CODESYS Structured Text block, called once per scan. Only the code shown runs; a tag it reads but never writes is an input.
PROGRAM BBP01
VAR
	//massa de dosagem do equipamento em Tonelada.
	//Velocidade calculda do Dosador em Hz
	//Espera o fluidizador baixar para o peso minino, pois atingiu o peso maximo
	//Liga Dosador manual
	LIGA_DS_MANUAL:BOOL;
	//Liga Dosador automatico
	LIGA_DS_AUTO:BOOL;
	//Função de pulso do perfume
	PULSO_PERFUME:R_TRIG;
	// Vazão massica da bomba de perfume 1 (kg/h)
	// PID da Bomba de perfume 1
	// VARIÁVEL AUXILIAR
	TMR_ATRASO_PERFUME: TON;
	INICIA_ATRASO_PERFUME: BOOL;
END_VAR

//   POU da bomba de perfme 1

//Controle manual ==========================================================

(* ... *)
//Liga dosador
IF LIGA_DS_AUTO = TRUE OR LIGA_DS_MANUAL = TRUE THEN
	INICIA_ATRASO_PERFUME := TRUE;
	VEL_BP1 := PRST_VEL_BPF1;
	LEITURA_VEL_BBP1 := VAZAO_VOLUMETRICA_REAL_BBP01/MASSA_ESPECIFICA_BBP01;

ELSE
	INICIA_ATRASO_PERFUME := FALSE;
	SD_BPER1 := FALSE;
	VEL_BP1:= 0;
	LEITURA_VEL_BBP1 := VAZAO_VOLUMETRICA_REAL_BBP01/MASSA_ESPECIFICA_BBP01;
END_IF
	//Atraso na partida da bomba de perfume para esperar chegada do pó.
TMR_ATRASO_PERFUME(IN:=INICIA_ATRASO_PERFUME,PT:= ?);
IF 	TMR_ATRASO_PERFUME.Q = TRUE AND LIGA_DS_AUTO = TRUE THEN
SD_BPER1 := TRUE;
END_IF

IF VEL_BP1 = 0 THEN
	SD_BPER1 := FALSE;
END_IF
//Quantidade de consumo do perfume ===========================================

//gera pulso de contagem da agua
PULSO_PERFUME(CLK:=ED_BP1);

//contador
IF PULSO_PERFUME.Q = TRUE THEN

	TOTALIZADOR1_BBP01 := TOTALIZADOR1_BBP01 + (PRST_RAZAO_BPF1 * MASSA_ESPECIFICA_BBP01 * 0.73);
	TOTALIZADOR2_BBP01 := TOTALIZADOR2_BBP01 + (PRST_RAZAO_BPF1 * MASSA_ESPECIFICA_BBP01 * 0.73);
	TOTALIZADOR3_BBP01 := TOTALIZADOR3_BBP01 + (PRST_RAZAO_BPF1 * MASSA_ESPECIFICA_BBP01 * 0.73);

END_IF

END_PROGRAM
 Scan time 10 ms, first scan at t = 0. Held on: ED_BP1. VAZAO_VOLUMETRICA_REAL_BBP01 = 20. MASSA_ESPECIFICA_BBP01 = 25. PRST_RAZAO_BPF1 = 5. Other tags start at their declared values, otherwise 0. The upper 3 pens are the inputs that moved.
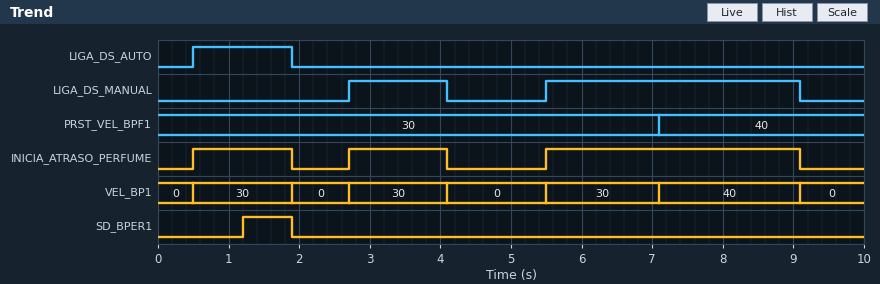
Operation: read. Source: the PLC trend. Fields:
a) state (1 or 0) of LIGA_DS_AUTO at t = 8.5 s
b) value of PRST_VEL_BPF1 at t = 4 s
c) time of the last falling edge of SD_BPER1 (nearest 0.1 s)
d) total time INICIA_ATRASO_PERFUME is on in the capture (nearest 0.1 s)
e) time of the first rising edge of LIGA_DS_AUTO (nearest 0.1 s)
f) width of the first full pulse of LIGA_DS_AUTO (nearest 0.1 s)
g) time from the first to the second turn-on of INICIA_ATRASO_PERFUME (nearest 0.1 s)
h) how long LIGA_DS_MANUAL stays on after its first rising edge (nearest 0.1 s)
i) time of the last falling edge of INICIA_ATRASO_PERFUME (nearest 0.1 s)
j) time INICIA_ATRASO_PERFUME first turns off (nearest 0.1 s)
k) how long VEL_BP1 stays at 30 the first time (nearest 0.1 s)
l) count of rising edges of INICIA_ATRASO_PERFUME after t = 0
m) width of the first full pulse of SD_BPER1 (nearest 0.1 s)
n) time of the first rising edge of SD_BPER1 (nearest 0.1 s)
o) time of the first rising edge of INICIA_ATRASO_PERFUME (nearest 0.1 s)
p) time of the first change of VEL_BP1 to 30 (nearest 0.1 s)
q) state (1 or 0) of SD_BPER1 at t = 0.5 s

0
30
1.9 s
6.4 s
0.5 s
1.4 s
2.2 s
1.4 s
9.1 s
1.9 s
1.4 s
3
0.7 s
1.2 s
0.5 s
0.5 s
0
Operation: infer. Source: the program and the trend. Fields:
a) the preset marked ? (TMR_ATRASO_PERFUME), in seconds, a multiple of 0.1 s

0.7 s
